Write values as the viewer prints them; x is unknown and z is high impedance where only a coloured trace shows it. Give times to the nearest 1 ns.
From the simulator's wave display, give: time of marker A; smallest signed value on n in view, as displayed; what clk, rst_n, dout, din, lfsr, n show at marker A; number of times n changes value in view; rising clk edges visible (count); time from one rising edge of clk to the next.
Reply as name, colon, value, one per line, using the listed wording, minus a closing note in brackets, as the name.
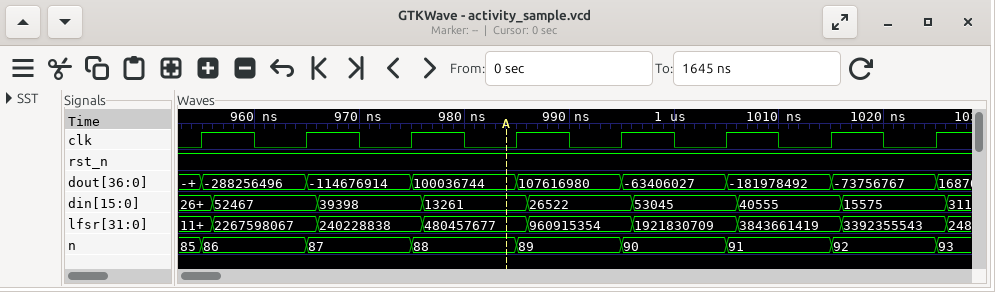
time of marker A: 984 ns
smallest signed value on n in view, as displayed: 85
what clk, rst_n, dout, din, lfsr, n show at marker A: clk=0, rst_n=1, dout=100036744, din=13261, lfsr=480457677, n=88
number of times n changes value in view: 8
rising clk edges visible: 8
time from one rising edge of clk to the next: 10 ns
